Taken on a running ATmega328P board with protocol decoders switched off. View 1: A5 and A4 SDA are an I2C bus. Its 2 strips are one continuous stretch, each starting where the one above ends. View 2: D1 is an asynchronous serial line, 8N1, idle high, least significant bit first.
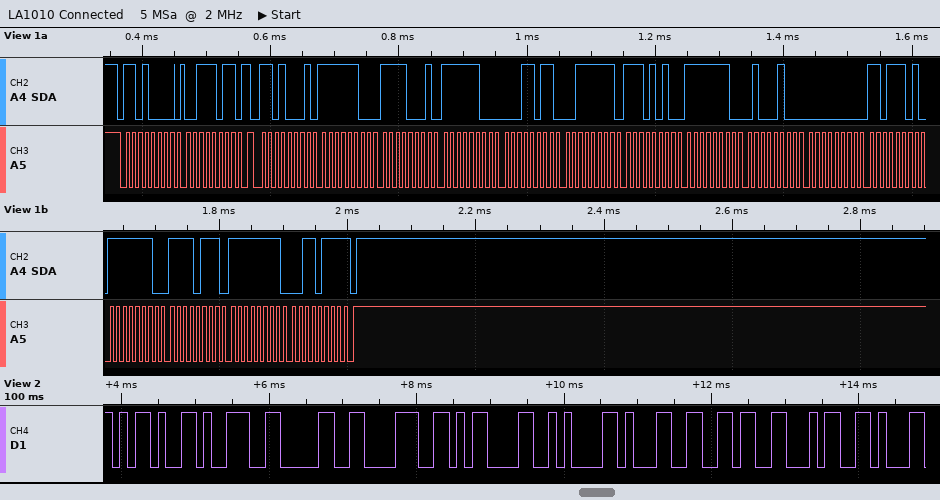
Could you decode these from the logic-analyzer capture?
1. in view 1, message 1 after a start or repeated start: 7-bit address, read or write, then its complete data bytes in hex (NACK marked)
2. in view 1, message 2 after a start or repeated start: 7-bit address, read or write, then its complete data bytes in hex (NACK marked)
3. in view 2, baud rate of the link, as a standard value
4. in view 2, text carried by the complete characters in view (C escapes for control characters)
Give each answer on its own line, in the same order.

0x68 write: 3B
0x68 read: FC F1 FC 1B 3F EA FE 44 00 DD FE F7 FF 37 NACK
9600 baud
"-908\r\n164"
